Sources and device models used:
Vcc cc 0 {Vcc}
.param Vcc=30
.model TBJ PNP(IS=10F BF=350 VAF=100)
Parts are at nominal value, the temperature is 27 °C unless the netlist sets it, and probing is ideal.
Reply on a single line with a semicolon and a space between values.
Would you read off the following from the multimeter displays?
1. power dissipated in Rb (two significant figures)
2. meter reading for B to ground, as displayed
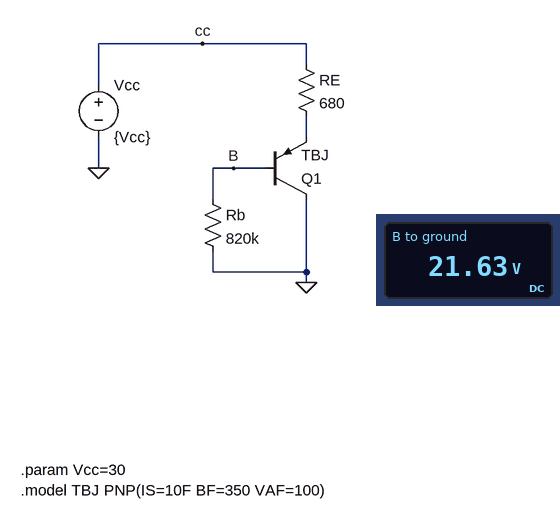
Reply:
570 µW; 21.63 V
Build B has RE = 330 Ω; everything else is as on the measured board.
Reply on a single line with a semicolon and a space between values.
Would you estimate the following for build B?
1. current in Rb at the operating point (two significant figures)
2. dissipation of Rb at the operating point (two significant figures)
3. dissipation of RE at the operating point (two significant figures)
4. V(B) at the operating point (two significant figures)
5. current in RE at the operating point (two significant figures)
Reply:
30 µA; 760 µW; 58 mW; 25 V; 13 mA
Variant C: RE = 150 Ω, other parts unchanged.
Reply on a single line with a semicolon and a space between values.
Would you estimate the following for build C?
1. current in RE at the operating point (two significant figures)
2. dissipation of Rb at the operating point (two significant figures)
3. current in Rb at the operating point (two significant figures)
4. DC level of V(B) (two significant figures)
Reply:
15 mA; 890 µW; 33 µA; 27 V
